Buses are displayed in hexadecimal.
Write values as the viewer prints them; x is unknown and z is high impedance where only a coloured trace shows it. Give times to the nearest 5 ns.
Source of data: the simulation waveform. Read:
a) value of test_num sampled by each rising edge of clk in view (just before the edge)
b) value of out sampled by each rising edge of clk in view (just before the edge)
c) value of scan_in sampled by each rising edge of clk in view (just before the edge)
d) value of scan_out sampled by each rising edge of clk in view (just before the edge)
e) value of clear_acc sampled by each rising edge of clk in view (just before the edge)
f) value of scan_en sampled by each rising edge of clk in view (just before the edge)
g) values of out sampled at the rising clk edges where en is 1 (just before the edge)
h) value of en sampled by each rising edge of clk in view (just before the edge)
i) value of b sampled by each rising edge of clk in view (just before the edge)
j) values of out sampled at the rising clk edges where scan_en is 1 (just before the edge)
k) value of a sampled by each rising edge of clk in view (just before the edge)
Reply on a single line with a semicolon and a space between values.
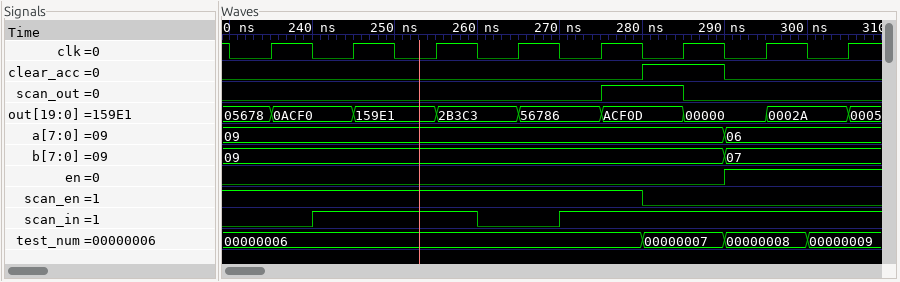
00000006, 00000006, 00000006, 00000006, 00000006, 00000007, 00000008, 00000009; 05678, 0ACF0, 159E1, 2B3C3, 56786, ACF0D, 00000, 0002A; 0 1 1 0 1 1 1 1; 0 0 0 0 0 1 0 0; 0 0 0 0 0 1 0 0; 1 1 1 1 1 0 0 0; 00000, 0002A; 0 0 0 0 0 0 1 1; 09, 09, 09, 09, 09, 09, 07, 07; 05678, 0ACF0, 159E1, 2B3C3, 56786; 09, 09, 09, 09, 09, 09, 06, 06
